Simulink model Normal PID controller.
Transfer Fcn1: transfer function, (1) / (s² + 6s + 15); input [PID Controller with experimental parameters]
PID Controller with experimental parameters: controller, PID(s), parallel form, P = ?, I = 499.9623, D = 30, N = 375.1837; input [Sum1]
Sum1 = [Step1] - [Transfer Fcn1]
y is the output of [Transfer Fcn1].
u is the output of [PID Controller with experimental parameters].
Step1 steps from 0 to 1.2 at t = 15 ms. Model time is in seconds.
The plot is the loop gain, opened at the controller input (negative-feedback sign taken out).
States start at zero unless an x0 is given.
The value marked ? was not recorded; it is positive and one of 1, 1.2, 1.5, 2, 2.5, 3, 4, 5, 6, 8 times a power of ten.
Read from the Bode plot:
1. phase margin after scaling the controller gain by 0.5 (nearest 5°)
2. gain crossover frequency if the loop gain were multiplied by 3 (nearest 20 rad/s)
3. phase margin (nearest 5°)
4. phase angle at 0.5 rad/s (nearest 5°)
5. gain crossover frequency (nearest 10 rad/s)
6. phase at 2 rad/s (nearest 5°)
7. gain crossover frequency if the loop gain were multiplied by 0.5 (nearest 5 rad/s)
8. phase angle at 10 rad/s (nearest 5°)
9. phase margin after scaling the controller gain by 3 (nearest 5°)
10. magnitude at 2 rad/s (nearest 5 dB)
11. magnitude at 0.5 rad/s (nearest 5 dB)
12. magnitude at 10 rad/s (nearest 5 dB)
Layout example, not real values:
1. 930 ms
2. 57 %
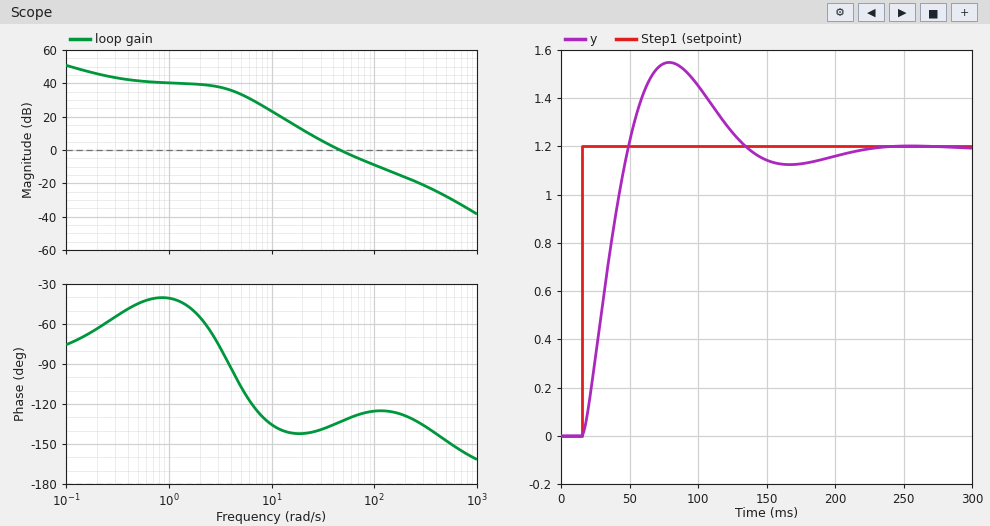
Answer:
1. 40°
2. 100 rad/s
3. 45°
4. -45°
5. 50 rad/s
6. -55°
7. 30 rad/s
8. -135°
9. 55°
10. 40 dB
11. 40 dB
12. 25 dB
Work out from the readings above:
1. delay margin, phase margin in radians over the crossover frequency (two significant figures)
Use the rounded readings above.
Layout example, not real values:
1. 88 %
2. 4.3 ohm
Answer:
1. 0.016 s
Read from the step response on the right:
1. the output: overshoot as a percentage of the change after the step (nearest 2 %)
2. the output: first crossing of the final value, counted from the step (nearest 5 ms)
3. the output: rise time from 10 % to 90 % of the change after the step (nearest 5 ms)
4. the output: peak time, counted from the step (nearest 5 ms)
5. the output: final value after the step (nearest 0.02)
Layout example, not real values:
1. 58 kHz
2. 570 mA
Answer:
1. 30 %
2. 35 ms
3. 25 ms
4. 65 ms
5. 1.20
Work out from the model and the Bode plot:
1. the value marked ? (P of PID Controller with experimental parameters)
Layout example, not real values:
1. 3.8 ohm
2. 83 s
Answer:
1. 1500
